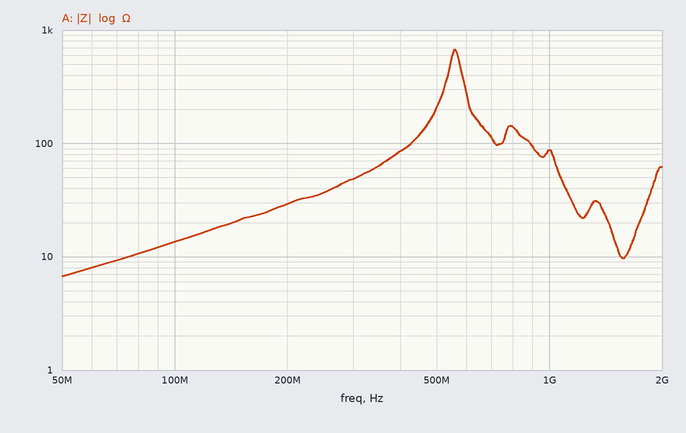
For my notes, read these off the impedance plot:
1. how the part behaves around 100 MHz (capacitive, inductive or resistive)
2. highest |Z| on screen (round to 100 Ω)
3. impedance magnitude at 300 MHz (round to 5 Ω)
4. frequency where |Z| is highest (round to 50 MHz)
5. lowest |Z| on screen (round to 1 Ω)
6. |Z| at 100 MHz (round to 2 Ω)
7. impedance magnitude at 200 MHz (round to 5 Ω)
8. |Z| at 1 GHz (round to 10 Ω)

inductive
700 Ω
50 Ω
550 MHz
7 Ω
14 Ω
30 Ω
90 Ω
